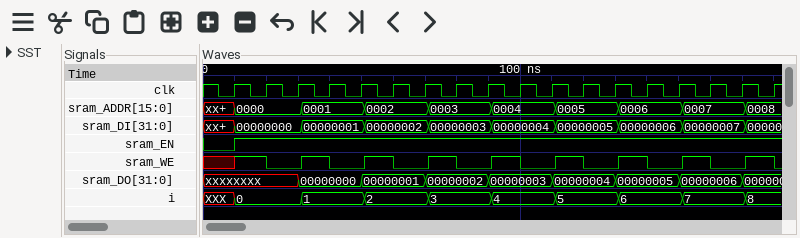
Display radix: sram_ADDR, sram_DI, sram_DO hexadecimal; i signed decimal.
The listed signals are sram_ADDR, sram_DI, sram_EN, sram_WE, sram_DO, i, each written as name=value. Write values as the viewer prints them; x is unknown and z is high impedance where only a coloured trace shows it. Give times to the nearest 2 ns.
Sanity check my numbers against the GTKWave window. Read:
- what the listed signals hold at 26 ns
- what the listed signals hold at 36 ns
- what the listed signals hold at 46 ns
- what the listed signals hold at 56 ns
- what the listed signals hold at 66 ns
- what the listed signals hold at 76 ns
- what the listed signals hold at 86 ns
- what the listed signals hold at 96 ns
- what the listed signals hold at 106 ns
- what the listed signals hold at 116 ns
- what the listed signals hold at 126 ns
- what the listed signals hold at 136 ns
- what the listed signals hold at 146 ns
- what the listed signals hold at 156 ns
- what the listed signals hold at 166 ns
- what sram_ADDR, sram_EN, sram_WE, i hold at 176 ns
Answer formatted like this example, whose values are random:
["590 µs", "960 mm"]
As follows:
["sram_ADDR=0000, sram_DI=00000000, sram_EN=1, sram_WE=0, sram_DO=xxxxxxxx, i=0", "sram_ADDR=0001, sram_DI=00000001, sram_EN=1, sram_WE=1, sram_DO=00000000, i=1", "sram_ADDR=0001, sram_DI=00000001, sram_EN=1, sram_WE=0, sram_DO=00000000, i=1", "sram_ADDR=0002, sram_DI=00000002, sram_EN=1, sram_WE=1, sram_DO=00000001, i=2", "sram_ADDR=0002, sram_DI=00000002, sram_EN=1, sram_WE=0, sram_DO=00000001, i=2", "sram_ADDR=0003, sram_DI=00000003, sram_EN=1, sram_WE=1, sram_DO=00000002, i=3", "sram_ADDR=0003, sram_DI=00000003, sram_EN=1, sram_WE=0, sram_DO=00000002, i=3", "sram_ADDR=0004, sram_DI=00000004, sram_EN=1, sram_WE=1, sram_DO=00000003, i=4", "sram_ADDR=0004, sram_DI=00000004, sram_EN=1, sram_WE=0, sram_DO=00000003, i=4", "sram_ADDR=0005, sram_DI=00000005, sram_EN=1, sram_WE=1, sram_DO=00000004, i=5", "sram_ADDR=0005, sram_DI=00000005, sram_EN=1, sram_WE=0, sram_DO=00000004, i=5", "sram_ADDR=0006, sram_DI=00000006, sram_EN=1, sram_WE=1, sram_DO=00000005, i=6", "sram_ADDR=0006, sram_DI=00000006, sram_EN=1, sram_WE=0, sram_DO=00000005, i=6", "sram_ADDR=0007, sram_DI=00000007, sram_EN=1, sram_WE=1, sram_DO=00000006, i=7", "sram_ADDR=0007, sram_DI=00000007, sram_EN=1, sram_WE=0, sram_DO=00000006, i=7", "sram_ADDR=0008, sram_EN=1, sram_WE=1, i=8"]
